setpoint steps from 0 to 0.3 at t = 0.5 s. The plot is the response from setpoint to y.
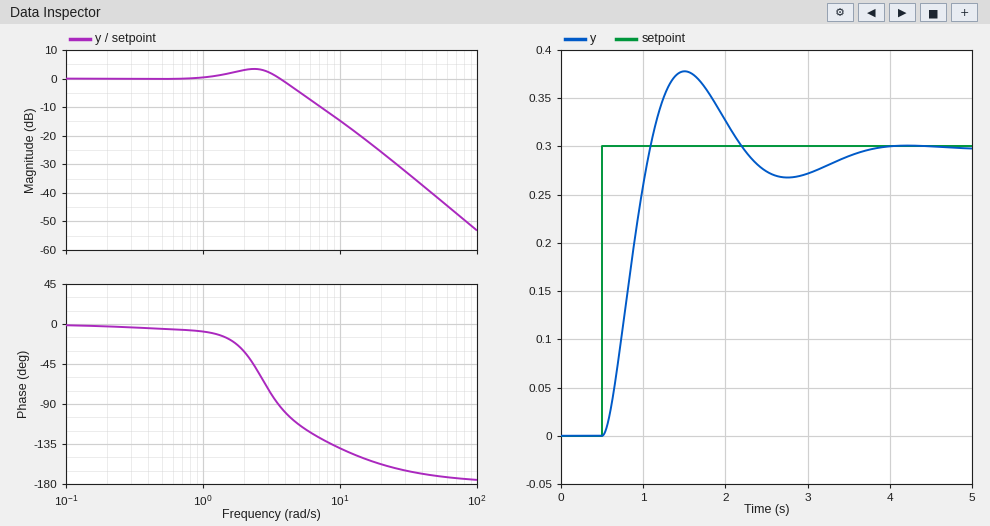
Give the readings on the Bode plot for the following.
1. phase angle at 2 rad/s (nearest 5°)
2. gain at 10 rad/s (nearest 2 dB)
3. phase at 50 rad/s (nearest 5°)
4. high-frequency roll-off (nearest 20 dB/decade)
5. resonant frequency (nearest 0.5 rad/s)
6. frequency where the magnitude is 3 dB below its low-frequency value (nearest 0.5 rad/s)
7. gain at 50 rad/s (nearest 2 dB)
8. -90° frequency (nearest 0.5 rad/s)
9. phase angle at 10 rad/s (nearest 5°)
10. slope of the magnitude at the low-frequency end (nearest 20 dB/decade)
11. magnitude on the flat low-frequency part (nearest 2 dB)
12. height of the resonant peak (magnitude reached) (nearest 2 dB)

-30°
-14 dB
-170°
-40 dB/decade
2.5 rad/s
4.5 rad/s
-42 dB
3.5 rad/s
-140°
0 dB/decade
0 dB
4 dB
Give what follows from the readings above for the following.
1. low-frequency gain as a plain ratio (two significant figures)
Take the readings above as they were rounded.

1.0
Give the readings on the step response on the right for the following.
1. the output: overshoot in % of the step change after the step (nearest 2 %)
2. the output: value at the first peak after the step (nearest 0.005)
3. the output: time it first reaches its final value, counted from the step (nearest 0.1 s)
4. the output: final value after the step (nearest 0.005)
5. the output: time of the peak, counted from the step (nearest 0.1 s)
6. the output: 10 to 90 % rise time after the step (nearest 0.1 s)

26 %
0.380
0.6 s
0.300
1.0 s
0.4 s
